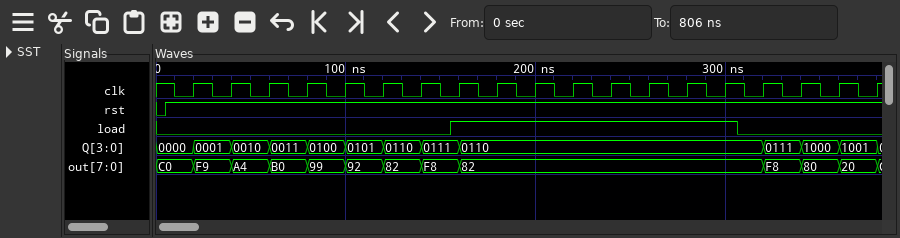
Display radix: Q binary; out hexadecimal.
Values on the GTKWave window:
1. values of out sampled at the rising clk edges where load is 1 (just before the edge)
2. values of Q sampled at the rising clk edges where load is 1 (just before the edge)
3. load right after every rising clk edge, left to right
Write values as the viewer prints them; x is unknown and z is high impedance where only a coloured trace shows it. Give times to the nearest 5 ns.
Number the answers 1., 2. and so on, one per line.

1. F8, 82, 82, 82, 82, 82, 82, 82
2. 0111, 0110, 0110, 0110, 0110, 0110, 0110, 0110
3. 0 0 0 0 0 0 0 1 1 1 1 1 1 1 1 0 0 0 0
